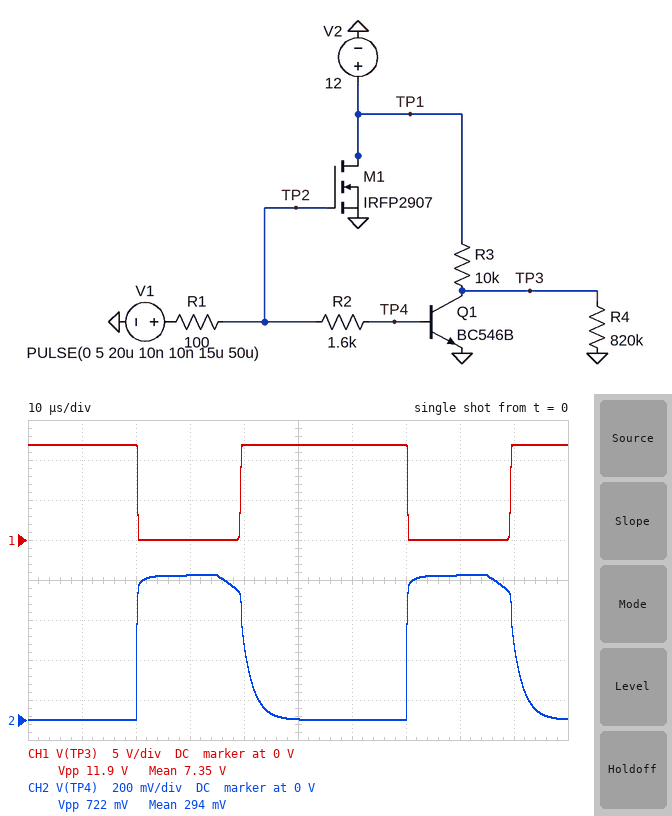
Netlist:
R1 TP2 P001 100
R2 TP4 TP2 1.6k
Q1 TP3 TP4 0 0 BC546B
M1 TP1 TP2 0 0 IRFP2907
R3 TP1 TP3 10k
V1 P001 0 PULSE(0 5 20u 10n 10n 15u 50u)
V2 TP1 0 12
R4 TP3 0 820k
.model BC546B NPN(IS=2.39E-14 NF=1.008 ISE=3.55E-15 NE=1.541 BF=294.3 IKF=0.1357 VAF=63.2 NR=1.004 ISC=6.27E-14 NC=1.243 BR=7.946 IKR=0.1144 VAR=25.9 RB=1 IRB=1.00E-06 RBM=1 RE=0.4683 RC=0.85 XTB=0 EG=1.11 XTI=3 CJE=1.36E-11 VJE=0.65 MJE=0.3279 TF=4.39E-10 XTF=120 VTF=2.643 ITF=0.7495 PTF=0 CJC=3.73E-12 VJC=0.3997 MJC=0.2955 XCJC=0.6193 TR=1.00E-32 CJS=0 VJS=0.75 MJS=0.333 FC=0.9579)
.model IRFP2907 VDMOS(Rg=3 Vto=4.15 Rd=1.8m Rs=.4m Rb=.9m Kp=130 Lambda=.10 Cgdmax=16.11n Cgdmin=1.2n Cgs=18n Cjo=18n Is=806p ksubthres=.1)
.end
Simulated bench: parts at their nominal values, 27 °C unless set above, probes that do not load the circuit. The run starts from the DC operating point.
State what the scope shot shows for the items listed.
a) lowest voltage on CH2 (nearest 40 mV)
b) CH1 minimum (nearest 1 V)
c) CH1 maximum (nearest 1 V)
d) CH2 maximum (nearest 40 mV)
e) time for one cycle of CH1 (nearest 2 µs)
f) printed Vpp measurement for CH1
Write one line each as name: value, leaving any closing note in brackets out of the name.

lowest voltage on CH2: 0 V
CH1 minimum: 0 V
CH1 maximum: 12 V
CH2 maximum: 720 mV
time for one cycle of CH1: 50 µs
printed Vpp measurement for CH1: 11.9 V
